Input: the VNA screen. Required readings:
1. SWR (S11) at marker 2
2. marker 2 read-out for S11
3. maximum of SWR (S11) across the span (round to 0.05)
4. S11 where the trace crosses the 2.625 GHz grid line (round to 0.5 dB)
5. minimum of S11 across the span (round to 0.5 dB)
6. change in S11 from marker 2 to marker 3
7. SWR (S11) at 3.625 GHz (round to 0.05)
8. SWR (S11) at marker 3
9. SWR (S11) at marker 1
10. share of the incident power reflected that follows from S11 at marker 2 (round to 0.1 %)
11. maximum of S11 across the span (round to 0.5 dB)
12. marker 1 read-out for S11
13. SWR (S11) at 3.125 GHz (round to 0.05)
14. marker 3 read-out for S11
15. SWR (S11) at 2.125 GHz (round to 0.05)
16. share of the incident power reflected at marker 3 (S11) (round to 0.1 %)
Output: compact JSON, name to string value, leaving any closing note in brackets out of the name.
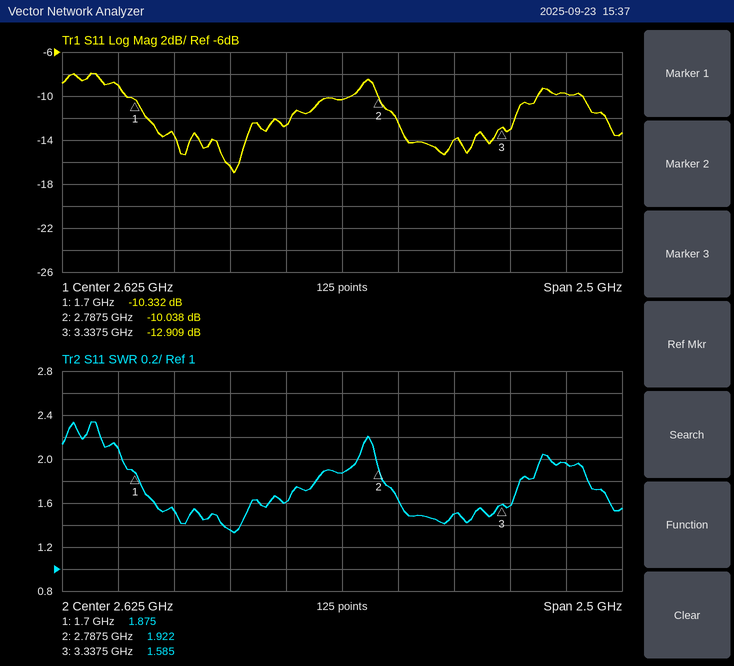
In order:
{"SWR (S11) at marker 2": "1.922", "marker 2 read-out for S11": "-10.038 dB", "maximum of SWR (S11) across the span": "2.35", "S11 where the trace crosses the 2.625 GHz grid line": "-10.5 dB", "minimum of S11 across the span": "-17.0 dB", "change in S11 from marker 2 to marker 3": "-2.871 dB", "SWR (S11) at 3.625 GHz": "1.95", "SWR (S11) at marker 3": "1.585", "SWR (S11) at marker 1": "1.875", "share of the incident power reflected that follows from S11 at marker 2": "9.9 %", "maximum of S11 across the span": "-8.0 dB", "marker 1 read-out for S11": "-10.332 dB", "SWR (S11) at 3.125 GHz": "1.50", "marker 3 read-out for S11": "-12.909 dB", "SWR (S11) at 2.125 GHz": "1.35", "share of the incident power reflected at marker 3 (S11)": "5.1 %"}
